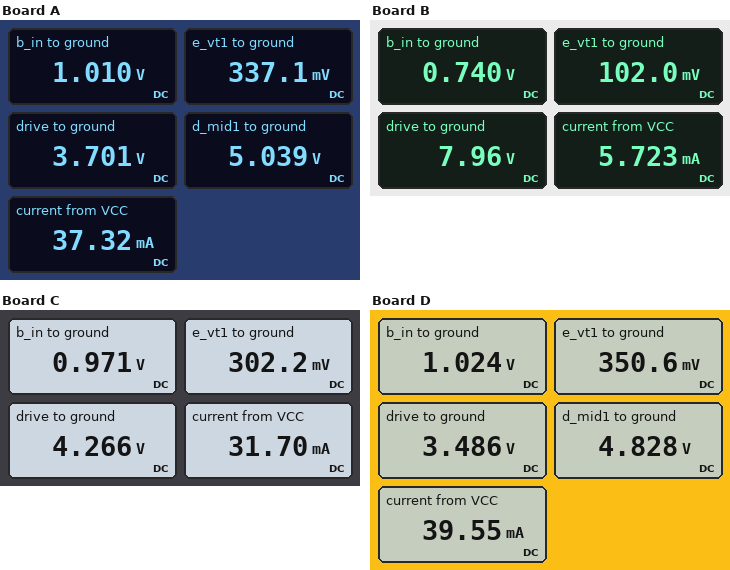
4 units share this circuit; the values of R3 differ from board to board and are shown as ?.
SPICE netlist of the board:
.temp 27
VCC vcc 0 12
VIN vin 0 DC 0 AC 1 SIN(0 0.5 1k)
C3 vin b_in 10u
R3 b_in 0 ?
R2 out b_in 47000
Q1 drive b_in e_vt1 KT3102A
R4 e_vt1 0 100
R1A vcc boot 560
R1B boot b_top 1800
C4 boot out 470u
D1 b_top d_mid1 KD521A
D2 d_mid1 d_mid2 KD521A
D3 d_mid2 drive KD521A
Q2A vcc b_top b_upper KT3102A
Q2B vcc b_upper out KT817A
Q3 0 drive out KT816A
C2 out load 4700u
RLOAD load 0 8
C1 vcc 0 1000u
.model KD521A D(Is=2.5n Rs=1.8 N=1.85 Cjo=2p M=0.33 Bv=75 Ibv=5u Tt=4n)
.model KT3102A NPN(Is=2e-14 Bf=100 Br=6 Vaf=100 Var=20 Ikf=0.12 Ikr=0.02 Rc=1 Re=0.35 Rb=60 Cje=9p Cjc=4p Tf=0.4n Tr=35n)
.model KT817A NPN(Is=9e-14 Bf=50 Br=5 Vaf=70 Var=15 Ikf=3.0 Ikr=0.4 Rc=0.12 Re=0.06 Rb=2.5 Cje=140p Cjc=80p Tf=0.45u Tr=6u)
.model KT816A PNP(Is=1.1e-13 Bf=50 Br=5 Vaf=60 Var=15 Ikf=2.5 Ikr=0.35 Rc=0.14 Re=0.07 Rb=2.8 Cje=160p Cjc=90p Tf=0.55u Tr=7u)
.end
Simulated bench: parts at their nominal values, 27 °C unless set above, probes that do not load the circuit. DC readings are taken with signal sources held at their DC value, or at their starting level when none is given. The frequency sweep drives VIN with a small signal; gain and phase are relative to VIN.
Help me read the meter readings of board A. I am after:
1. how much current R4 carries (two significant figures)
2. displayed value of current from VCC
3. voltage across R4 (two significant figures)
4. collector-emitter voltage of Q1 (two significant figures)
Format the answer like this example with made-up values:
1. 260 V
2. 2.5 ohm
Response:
1. 3.4 mA
2. 37.32 mA
3. 340 mV
4. 3.4 V
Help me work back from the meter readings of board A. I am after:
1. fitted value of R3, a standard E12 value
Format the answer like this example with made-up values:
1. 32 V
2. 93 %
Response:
1. 27 kΩ
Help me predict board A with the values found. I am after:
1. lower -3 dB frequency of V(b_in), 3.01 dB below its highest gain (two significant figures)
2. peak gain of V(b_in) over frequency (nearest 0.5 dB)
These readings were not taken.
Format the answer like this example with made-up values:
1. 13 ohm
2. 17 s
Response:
1. 3.5 Hz
2. 0 dB
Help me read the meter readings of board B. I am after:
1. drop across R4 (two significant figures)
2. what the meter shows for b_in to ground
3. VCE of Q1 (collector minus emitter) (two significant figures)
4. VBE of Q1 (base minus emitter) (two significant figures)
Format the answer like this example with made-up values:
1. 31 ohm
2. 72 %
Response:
1. 100 mV
2. 0.740 V
3. 7.9 V
4. 640 mV
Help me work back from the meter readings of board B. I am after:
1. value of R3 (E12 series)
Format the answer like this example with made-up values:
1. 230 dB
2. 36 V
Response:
1. 4.7 kΩ
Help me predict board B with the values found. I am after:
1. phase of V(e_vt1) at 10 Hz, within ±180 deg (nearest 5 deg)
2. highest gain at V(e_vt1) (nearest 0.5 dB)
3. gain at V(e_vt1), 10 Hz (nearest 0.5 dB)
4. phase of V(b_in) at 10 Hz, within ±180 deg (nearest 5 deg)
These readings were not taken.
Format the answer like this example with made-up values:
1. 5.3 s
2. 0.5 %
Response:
1. 35 deg
2. -2.0 dB
3. -3.0 dB
4. 35 deg
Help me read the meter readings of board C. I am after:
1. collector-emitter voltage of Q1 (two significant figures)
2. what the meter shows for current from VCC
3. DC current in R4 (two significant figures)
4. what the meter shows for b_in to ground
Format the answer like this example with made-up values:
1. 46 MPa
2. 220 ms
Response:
1. 4.0 V
2. 31.70 mA
3. 3.0 mA
4. 0.971 V
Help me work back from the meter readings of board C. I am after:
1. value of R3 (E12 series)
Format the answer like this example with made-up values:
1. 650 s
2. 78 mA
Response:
1. 18 kΩ
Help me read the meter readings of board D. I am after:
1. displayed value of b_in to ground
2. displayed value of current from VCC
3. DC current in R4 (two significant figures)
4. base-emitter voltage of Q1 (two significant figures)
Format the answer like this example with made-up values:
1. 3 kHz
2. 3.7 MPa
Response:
1. 1.024 V
2. 39.55 mA
3. 3.5 mA
4. 670 mV
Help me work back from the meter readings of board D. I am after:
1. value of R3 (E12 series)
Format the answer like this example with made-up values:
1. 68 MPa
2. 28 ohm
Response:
1. 33 kΩ
